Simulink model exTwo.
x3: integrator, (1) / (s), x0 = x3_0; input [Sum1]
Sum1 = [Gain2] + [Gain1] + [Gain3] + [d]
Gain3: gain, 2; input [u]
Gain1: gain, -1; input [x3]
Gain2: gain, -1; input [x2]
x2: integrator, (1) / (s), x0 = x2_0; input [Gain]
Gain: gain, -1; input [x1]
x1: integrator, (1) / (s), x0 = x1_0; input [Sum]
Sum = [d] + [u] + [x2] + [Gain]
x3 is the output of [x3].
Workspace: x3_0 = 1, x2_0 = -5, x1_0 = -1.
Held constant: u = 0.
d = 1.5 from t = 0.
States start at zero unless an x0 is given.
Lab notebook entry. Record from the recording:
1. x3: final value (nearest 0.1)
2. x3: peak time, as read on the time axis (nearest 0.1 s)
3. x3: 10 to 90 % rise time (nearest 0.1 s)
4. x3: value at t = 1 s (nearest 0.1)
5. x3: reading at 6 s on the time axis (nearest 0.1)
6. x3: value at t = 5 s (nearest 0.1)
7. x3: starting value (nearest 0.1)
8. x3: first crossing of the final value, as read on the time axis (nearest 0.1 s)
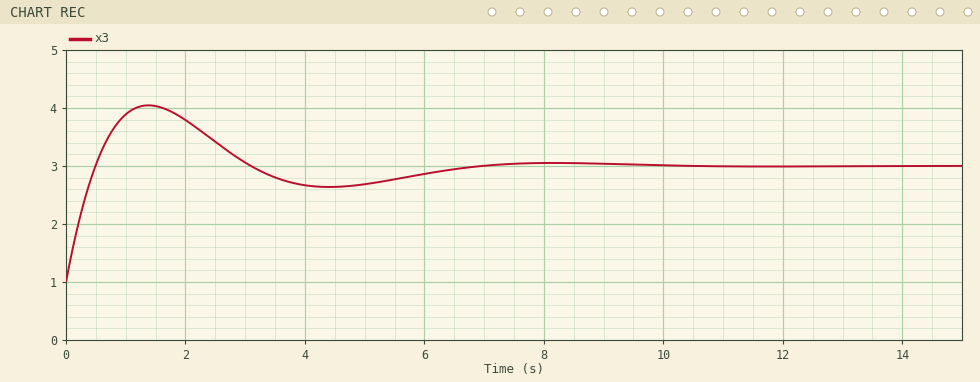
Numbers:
3.0
1.4 s
0.4 s
3.9
2.9
2.7
1.0
0.5 s
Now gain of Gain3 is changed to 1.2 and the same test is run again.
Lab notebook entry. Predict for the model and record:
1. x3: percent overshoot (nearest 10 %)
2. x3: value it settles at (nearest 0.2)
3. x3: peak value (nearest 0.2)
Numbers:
50 %
3.0
4.0
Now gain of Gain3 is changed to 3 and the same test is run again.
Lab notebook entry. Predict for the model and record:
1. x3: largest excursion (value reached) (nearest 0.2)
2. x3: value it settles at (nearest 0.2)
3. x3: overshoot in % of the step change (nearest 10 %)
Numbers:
4.0
3.0
50 %
